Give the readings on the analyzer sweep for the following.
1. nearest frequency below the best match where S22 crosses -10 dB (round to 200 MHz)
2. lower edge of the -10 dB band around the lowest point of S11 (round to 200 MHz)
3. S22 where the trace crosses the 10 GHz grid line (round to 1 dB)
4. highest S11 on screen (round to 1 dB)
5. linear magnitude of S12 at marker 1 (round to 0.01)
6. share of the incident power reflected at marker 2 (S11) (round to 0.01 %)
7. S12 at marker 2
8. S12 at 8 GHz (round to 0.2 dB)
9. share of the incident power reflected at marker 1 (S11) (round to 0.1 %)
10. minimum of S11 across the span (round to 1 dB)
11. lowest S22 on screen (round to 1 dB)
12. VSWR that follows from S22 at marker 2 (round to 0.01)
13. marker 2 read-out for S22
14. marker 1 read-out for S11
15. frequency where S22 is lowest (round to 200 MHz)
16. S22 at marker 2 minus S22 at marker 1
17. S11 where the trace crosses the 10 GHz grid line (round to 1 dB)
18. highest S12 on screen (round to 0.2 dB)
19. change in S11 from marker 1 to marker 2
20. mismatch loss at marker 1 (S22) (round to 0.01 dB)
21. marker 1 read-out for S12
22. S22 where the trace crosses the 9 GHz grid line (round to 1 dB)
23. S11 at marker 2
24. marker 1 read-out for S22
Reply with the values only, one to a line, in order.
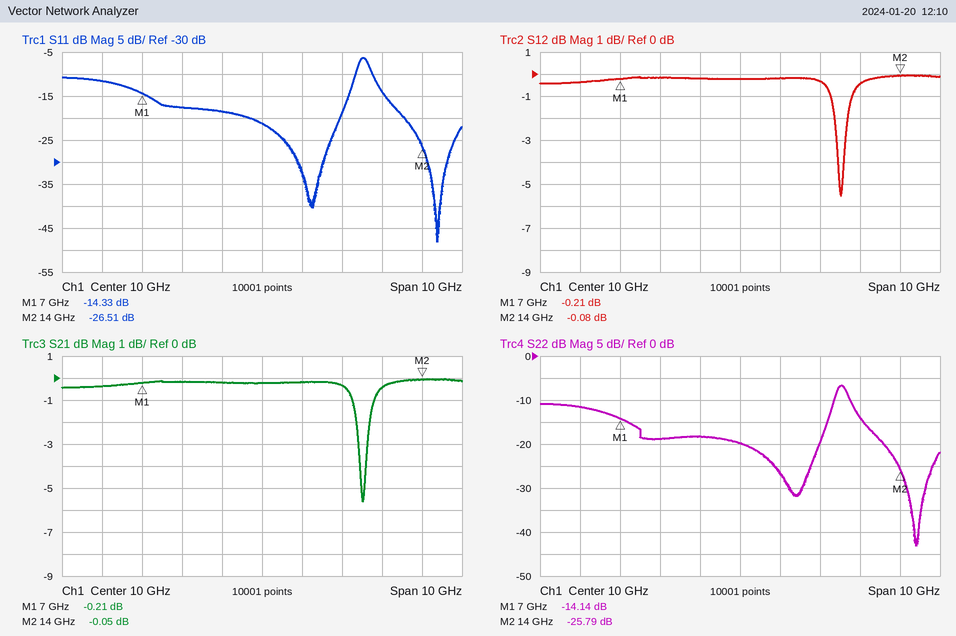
12.8 GHz
12.8 GHz
-20 dB
-6 dB
0.98
0.22 %
-0.08 dB
-0.2 dB
3.7 %
-48 dB
-43 dB
1.11
-25.79 dB
-14.33 dB
14.4 GHz
-11.65 dB
-21 dB
0.0 dB
-12.18 dB
0.17 dB
-0.21 dB
-18 dB
-26.51 dB
-14.14 dB
